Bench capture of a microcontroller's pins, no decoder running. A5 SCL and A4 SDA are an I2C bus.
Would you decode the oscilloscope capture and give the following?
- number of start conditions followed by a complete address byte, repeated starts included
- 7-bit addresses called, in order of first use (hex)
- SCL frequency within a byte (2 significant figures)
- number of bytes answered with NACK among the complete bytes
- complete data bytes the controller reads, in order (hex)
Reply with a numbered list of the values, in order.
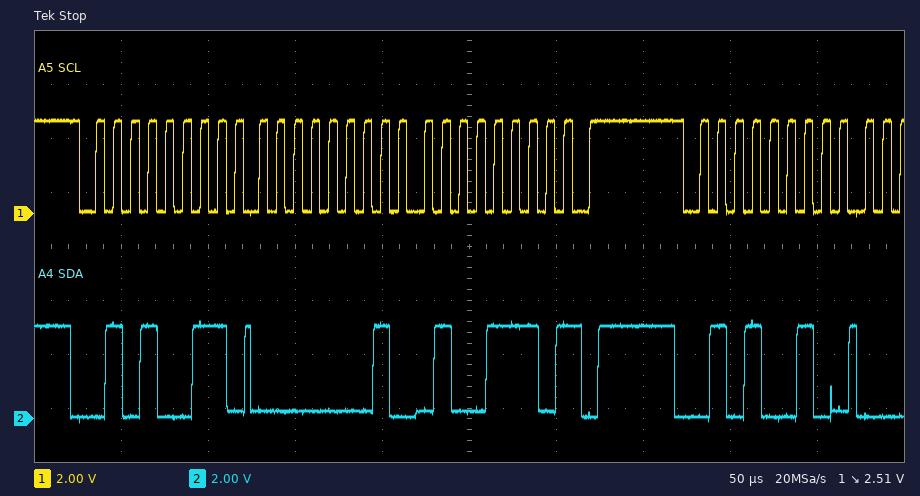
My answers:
1. 2
2. 0x29
3. 100 kHz
4. 1
5. 01 4E
